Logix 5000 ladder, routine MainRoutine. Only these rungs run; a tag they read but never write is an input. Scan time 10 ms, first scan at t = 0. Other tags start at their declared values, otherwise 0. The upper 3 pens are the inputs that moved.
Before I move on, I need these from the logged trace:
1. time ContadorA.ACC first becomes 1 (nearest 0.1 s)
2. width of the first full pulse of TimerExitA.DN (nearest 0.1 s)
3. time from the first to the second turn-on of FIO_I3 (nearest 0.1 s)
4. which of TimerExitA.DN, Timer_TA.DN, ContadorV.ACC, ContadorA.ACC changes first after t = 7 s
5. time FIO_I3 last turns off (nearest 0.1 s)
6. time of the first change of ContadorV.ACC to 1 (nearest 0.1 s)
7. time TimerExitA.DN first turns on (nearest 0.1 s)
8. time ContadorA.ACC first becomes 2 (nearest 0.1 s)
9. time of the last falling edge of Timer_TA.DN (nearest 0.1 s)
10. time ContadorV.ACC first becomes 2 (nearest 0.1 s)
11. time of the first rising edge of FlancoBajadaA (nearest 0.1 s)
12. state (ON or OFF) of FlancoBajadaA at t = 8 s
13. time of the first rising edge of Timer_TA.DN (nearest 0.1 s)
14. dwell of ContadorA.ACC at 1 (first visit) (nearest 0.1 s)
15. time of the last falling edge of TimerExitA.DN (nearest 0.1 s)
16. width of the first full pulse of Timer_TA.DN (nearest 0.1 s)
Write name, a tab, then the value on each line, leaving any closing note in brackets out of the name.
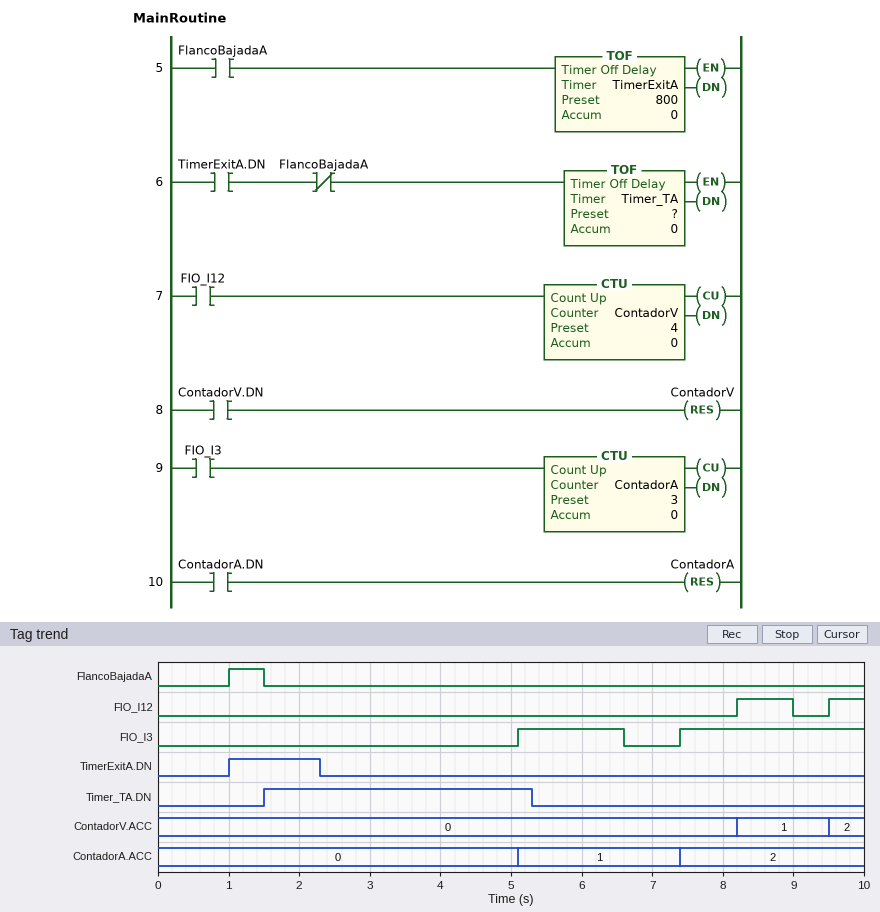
time ContadorA.ACC first becomes 1	5.1 s
width of the first full pulse of TimerExitA.DN	1.3 s
time from the first to the second turn-on of FIO_I3	2.3 s
which of TimerExitA.DN, Timer_TA.DN, ContadorV.ACC, ContadorA.ACC changes first after t = 7 s	ContadorA.ACC
time FIO_I3 last turns off	6.6 s
time of the first change of ContadorV.ACC to 1	8.2 s
time TimerExitA.DN first turns on	1.0 s
time ContadorA.ACC first becomes 2	7.4 s
time of the last falling edge of Timer_TA.DN	5.3 s
time ContadorV.ACC first becomes 2	9.5 s
time of the first rising edge of FlancoBajadaA	1.0 s
state (ON or OFF) of FlancoBajadaA at t = 8 s	OFF
time of the first rising edge of Timer_TA.DN	1.5 s
dwell of ContadorA.ACC at 1 (first visit)	2.3 s
time of the last falling edge of TimerExitA.DN	2.3 s
width of the first full pulse of Timer_TA.DN	3.8 s
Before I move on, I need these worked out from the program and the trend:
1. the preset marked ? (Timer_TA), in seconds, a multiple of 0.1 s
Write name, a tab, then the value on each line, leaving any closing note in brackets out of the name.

the preset marked ? (Timer_TA), in seconds, a multiple of 0.1 s	3.0 s
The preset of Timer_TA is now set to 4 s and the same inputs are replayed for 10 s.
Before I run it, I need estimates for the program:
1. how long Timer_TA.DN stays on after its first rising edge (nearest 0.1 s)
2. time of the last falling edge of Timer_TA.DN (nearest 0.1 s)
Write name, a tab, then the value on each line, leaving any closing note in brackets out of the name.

how long Timer_TA.DN stays on after its first rising edge	4.8 s
time of the last falling edge of Timer_TA.DN	6.3 s
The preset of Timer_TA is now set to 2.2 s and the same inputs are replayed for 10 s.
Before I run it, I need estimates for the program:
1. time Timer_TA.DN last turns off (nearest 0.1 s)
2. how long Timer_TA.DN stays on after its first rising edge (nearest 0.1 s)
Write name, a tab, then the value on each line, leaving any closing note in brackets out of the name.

time Timer_TA.DN last turns off	4.5 s
how long Timer_TA.DN stays on after its first rising edge	3.0 s
